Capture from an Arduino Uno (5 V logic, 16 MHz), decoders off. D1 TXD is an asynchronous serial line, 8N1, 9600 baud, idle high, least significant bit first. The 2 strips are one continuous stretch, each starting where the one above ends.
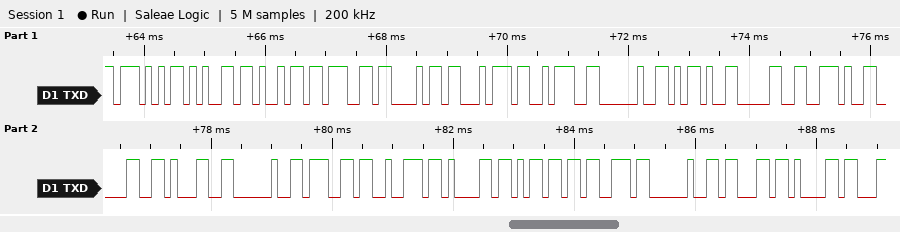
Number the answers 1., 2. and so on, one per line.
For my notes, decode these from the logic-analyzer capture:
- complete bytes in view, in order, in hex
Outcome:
1. 57 65 69 67 68 74 3A 20 2D 30 2E 30 31 20 67 72 61 6D 73 20 63 61
